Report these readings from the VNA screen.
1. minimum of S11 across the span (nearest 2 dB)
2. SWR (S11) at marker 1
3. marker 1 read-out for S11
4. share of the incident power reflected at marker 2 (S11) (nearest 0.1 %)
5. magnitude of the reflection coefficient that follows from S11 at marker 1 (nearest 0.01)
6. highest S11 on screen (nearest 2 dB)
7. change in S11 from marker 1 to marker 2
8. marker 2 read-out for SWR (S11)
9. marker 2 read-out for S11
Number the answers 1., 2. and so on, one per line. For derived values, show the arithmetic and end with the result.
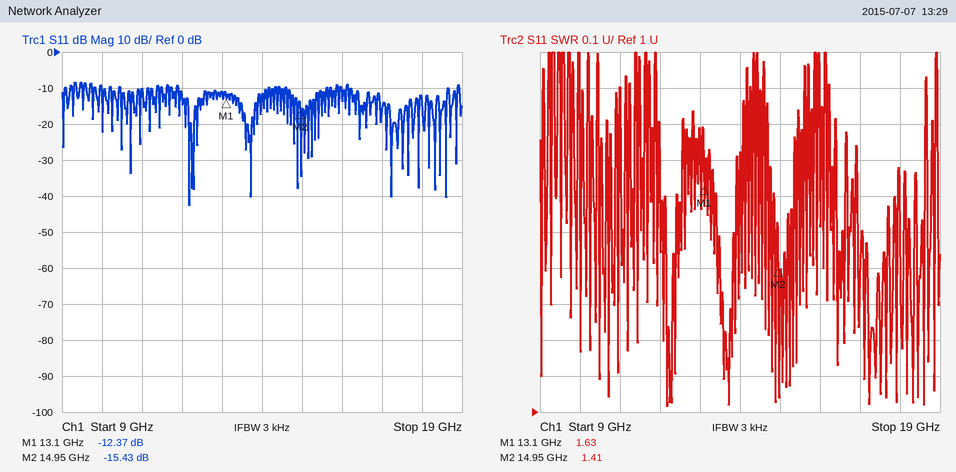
1. -42 dB
2. 1.63
3. -12.37 dB
4. 10^(-15.43/10) ≈ 2.9 %
5. 10^(-12.37/20) ≈ 0.24
6. -8 dB
7. -15.43 − (-12.37) = -3.06 dB
8. 1.41
9. -15.43 dB
